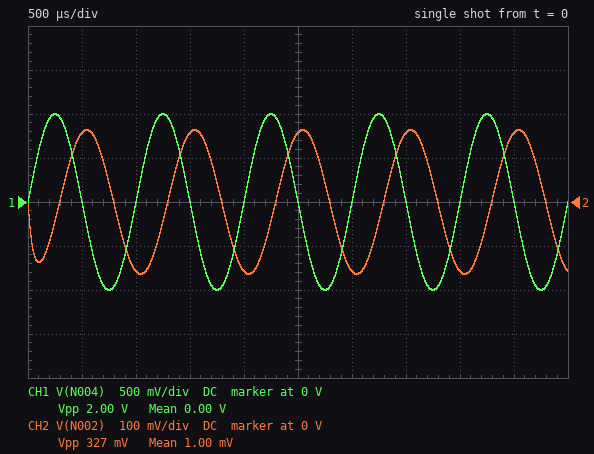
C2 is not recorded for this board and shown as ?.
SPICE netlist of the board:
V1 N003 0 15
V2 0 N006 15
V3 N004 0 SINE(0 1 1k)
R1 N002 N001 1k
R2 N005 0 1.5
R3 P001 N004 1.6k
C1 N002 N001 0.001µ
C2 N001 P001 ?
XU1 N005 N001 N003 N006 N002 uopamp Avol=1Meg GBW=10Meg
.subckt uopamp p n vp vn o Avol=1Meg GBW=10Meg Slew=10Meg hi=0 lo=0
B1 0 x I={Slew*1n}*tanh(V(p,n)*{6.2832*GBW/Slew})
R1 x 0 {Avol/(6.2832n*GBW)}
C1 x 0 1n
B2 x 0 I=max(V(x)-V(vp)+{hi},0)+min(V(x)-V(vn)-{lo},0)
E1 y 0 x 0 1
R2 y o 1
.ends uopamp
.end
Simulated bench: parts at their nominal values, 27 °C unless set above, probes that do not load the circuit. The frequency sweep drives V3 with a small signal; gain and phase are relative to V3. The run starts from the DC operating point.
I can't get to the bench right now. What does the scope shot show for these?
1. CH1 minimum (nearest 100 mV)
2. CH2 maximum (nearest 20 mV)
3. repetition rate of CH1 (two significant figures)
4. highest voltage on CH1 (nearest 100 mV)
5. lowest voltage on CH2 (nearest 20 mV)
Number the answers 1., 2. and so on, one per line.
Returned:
1. -1.0 V
2. 160 mV
3. 1.0 kHz
4. 1.0 V
5. -160 mV
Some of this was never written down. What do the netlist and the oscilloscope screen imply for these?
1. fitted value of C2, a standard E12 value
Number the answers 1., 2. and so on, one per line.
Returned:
1. 27 nF
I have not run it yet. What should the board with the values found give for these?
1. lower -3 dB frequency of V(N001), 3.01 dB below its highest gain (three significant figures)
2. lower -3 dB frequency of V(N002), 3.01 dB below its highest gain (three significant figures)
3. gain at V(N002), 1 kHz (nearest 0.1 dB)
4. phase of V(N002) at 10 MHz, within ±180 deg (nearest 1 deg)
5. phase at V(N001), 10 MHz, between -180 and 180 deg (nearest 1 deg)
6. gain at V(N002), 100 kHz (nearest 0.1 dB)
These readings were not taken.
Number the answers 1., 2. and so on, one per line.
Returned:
1. 153 kHz
2. 3.52 kHz
3. -15.7 dB
4. 46 deg
5. -40 deg
6. -5.6 dB
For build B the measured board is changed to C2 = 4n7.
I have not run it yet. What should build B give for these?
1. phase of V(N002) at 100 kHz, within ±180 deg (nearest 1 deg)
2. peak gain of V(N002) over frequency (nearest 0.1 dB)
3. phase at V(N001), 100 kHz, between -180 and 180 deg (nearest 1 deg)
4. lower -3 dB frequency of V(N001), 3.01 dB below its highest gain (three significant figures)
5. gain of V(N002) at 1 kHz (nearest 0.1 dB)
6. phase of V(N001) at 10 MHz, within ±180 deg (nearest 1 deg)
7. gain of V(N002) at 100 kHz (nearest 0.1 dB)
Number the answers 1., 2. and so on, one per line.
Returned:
1. 159 deg
2. -5.2 dB
3. 69 deg
4. 155 kHz
5. -30.6 dB
6. -40 deg
7. -5.7 dB
